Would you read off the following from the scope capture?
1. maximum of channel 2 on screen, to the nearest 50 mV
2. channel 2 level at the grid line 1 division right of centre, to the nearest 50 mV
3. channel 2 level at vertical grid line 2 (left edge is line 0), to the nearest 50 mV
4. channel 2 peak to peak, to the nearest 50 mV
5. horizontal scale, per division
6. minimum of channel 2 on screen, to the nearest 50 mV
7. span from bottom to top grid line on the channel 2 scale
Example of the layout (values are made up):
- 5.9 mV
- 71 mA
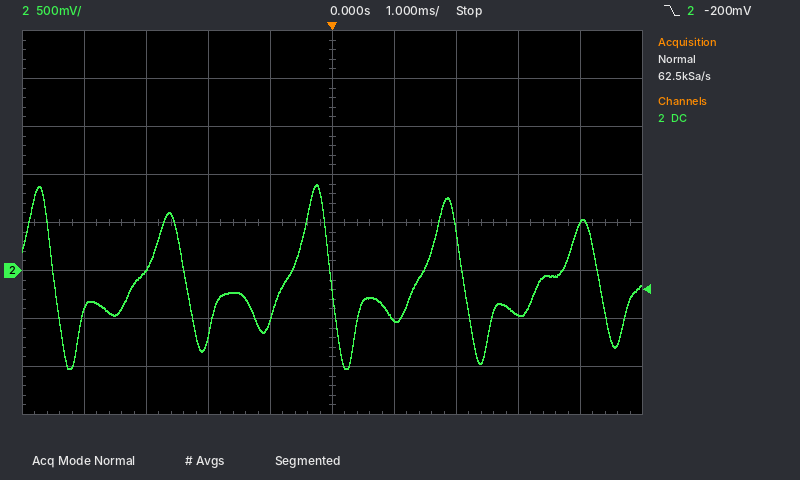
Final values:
- 900 mV
- -500 mV
- 0 mV
- 1.90 V
- 1 ms
- -1.00 V
- 4 V
